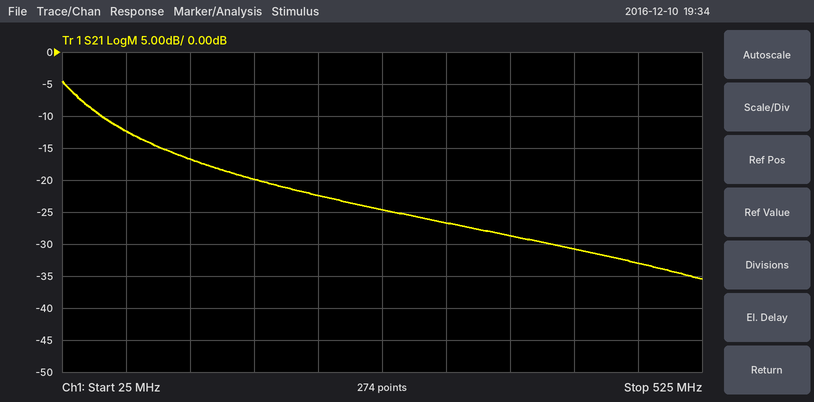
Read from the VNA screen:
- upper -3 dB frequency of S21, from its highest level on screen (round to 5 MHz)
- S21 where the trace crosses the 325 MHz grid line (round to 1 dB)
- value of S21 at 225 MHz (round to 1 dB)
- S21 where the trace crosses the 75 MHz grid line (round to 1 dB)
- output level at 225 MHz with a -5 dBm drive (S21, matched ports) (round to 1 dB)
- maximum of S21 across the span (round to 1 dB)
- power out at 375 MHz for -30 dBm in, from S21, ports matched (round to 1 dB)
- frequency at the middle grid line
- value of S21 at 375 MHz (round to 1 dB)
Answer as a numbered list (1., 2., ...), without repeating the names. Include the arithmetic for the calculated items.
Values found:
1. 40 MHz
2. -27 dB
3. -22 dB
4. -12 dB
5. -5 dBm + (-22 dB) = -27 dBm
6. -5 dB
7. -30 dBm + (-29 dB) = -59 dBm
8. 275 MHz
9. -29 dB
